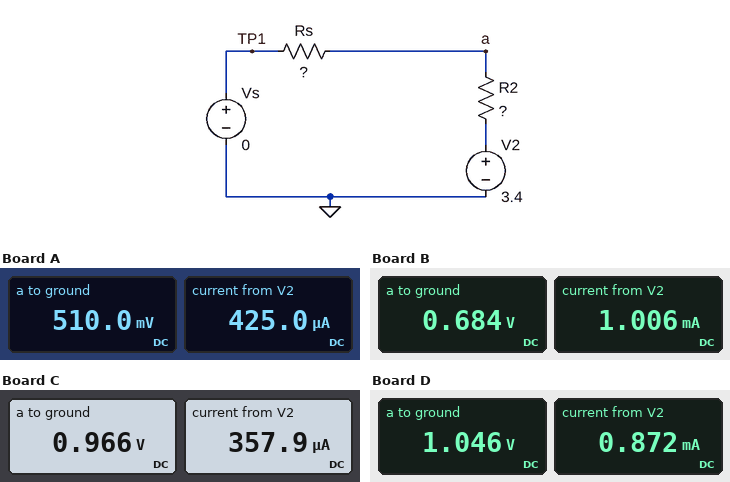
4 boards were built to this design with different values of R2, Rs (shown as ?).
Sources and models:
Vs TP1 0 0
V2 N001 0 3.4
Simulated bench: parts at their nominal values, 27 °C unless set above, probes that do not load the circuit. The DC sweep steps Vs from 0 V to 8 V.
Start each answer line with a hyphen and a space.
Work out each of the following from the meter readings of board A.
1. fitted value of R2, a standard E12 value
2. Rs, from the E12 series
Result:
- 6.8 kΩ
- 1.2 kΩ
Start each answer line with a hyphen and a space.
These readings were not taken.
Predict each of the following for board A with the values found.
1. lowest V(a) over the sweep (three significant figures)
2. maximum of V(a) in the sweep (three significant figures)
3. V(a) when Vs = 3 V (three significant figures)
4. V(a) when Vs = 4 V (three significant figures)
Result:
- 510 mV
- 7.31 V
- 3.06 V
- 3.91 V
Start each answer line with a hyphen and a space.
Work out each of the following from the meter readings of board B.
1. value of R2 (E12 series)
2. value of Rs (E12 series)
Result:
- 2.7 kΩ
- 680 Ω
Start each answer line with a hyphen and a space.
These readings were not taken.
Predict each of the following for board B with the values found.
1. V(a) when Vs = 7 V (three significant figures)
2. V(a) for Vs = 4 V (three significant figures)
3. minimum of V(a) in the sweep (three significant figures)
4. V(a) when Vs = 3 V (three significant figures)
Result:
- 6.28 V
- 3.88 V
- 684 mV
- 3.08 V
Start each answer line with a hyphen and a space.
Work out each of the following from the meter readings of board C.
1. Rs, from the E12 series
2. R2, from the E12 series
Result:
- 2.7 kΩ
- 6.8 kΩ
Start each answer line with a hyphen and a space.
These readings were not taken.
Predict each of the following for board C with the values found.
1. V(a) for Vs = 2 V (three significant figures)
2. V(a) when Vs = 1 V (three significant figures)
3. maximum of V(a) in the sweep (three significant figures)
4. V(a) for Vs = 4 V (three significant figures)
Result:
- 2.40 V
- 1.68 V
- 6.69 V
- 3.83 V
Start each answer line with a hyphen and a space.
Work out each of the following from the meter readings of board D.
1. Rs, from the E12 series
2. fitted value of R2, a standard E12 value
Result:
- 1.2 kΩ
- 2.7 kΩ
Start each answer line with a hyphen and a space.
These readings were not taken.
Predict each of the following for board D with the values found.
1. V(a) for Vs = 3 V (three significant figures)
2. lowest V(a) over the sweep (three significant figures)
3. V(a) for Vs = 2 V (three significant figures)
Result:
- 3.12 V
- 1.05 V
- 2.43 V
